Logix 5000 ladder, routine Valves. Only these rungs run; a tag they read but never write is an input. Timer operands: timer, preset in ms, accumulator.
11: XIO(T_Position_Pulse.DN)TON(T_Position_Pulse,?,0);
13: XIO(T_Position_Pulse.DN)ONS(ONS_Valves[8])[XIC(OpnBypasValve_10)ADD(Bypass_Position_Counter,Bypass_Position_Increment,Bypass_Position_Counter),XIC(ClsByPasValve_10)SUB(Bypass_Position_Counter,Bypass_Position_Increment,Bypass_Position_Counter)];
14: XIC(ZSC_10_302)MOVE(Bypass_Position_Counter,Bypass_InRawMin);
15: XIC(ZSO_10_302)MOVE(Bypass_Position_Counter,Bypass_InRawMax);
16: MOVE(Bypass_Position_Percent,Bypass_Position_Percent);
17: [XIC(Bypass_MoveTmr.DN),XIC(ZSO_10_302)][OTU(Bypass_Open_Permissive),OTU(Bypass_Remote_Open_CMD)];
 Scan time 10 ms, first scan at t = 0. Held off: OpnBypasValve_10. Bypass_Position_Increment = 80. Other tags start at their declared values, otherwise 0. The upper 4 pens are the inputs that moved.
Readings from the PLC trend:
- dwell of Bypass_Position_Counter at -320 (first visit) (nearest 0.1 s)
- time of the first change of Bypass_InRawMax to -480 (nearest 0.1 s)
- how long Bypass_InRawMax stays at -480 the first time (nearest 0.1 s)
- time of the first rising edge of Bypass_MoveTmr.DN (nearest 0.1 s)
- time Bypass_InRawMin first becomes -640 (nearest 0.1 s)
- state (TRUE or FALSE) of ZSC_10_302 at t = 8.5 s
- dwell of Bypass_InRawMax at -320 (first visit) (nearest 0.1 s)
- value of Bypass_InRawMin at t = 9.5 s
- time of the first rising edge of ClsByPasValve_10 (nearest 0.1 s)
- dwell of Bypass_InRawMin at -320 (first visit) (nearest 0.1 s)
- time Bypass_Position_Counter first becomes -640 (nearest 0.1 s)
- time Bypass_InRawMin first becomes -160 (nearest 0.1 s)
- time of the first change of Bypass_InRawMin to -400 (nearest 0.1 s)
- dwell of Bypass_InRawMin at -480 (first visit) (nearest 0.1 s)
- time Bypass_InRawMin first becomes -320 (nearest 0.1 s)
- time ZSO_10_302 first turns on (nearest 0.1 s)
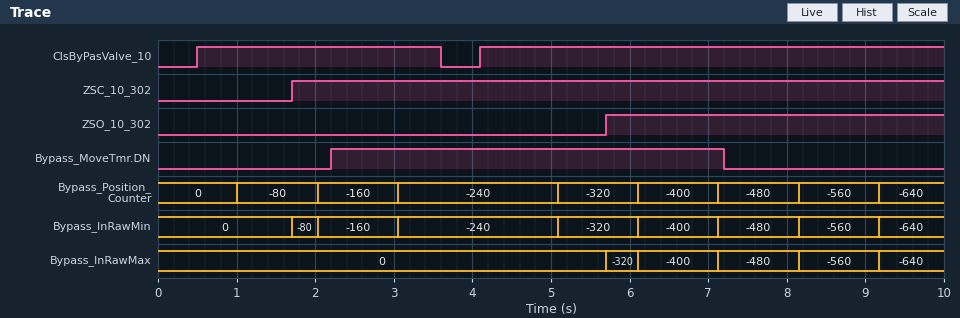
1.0 s
7.1 s
1.0 s
2.2 s
9.2 s
TRUE
0.4 s
-640
0.5 s
1.0 s
9.2 s
2.0 s
6.1 s
1.0 s
5.1 s
5.7 s
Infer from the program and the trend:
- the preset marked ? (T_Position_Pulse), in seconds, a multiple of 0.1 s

1.0 s
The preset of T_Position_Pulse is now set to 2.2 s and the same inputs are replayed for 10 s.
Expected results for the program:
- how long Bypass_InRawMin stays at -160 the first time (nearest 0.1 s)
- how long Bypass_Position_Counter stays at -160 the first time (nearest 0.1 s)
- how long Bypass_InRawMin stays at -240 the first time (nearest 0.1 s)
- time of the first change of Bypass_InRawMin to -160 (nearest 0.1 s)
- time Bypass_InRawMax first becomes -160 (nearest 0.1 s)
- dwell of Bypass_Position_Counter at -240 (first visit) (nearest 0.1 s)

2.2 s
2.2 s
2.2 s
4.4 s
5.7 s
2.2 s
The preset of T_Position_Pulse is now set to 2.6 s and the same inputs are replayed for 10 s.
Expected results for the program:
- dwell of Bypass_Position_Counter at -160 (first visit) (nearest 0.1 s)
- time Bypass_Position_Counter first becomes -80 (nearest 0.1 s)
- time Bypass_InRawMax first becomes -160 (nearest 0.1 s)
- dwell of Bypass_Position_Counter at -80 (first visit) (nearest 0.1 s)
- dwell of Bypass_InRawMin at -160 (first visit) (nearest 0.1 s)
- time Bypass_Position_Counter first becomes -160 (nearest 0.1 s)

2.6 s
2.6 s
5.7 s
2.6 s
2.6 s
5.2 s
